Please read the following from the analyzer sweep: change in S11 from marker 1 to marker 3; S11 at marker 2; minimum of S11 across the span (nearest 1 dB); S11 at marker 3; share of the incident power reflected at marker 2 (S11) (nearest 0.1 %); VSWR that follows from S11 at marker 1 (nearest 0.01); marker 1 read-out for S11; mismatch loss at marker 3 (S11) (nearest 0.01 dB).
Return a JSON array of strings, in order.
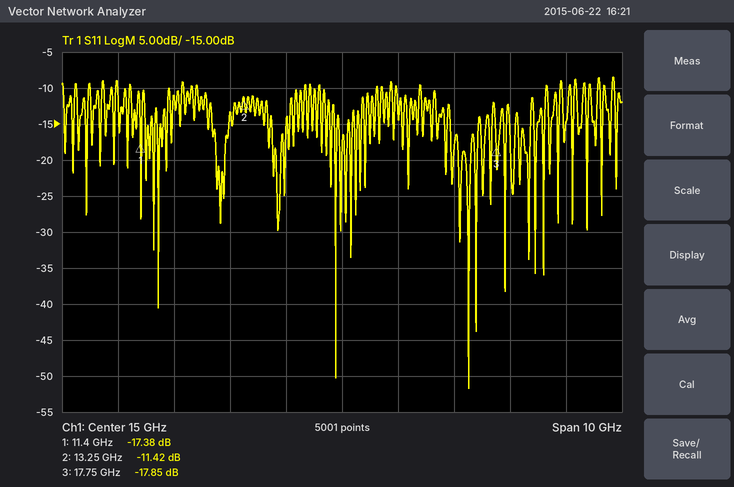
["-0.47 dB", "-11.42 dB", "-52 dB", "-17.85 dB", "7.2 %", "1.31", "-17.38 dB", "0.07 dB"]
